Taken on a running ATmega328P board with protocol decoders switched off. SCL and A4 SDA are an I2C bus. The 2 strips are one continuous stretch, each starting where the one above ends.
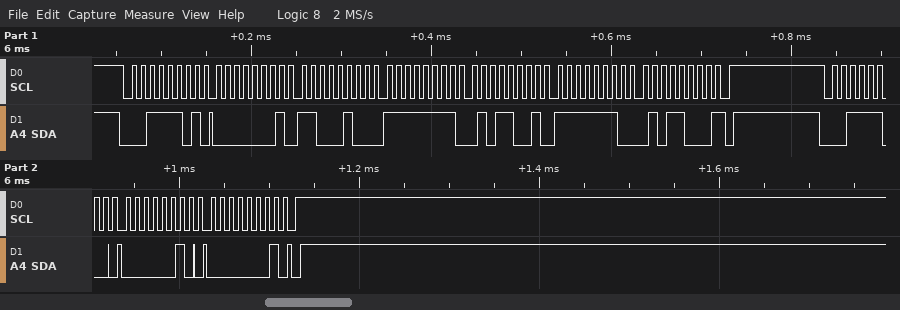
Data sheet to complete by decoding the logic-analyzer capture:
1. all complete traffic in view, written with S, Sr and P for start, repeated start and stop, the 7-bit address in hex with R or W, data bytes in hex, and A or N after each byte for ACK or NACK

S 1ER A 01 A C4 A FF A 59 A FE A 58 N P S 1EW A 02 A 01 A P
